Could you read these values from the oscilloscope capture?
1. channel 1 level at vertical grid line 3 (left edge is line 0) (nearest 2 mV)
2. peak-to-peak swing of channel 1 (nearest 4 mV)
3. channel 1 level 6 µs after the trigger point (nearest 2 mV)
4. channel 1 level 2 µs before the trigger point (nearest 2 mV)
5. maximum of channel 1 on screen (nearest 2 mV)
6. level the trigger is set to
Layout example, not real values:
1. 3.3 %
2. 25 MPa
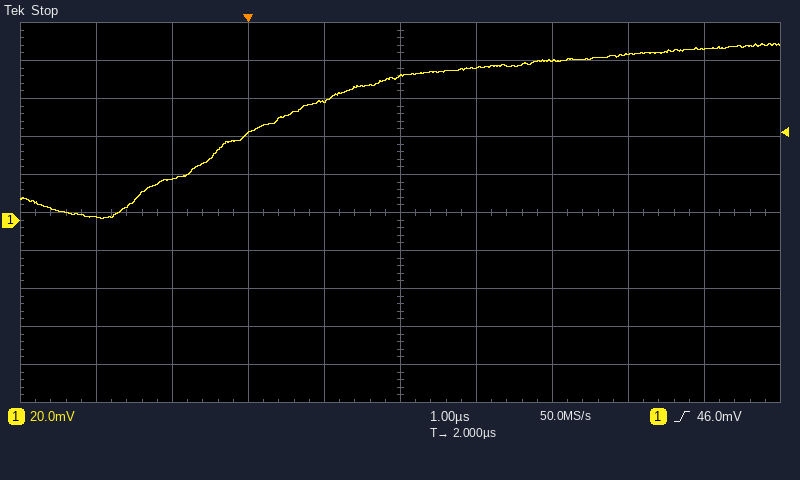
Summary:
1. 46 mV
2. 92 mV
3. 90 mV
4. 2 mV
5. 92 mV
6. 46.0 mV
